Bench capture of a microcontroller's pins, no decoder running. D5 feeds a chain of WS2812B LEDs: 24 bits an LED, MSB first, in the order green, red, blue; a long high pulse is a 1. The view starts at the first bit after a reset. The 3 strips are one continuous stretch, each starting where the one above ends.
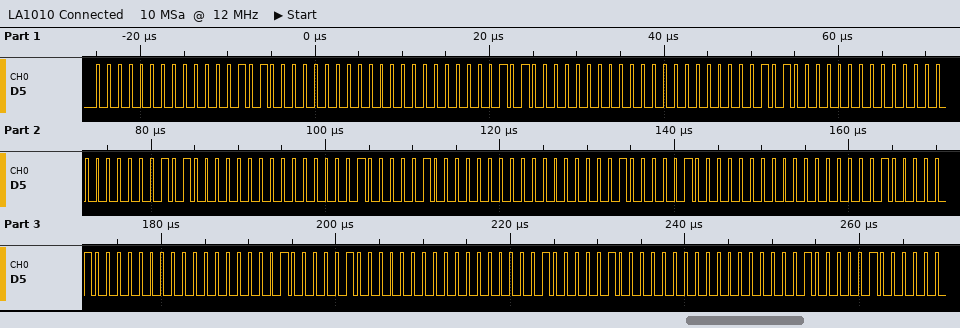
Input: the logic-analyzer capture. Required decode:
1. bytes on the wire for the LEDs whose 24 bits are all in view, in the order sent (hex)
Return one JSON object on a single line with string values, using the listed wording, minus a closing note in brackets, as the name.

{"bytes on the wire for the LEDs whose 24 bits are all in view, in the order sent": "00 05 00 00 05 00 00 05 00 00 05 00 01 04 00 01 04 00 01 04 00 01 04 00 01 04 00"}
